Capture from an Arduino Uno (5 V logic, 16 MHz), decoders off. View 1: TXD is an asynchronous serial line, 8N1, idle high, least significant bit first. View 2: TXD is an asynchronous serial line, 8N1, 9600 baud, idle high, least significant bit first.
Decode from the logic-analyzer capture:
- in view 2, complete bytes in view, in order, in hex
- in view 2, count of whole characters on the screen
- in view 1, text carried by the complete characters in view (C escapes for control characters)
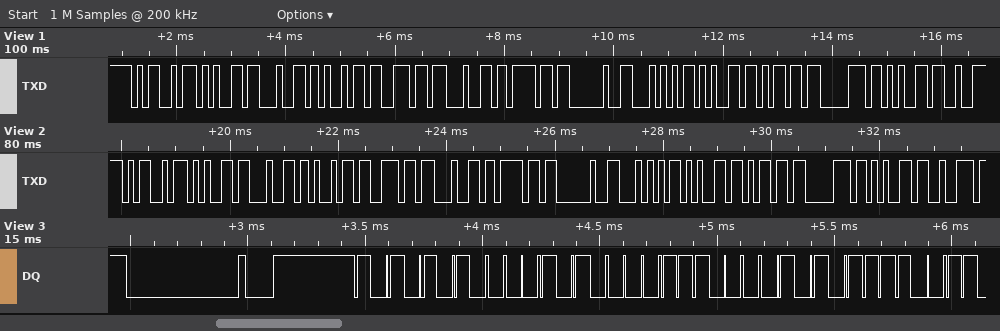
4D 65 64 69 6E 64 6F 20 54 65 6D 70 65 72
14
"Medindo Tempe"
